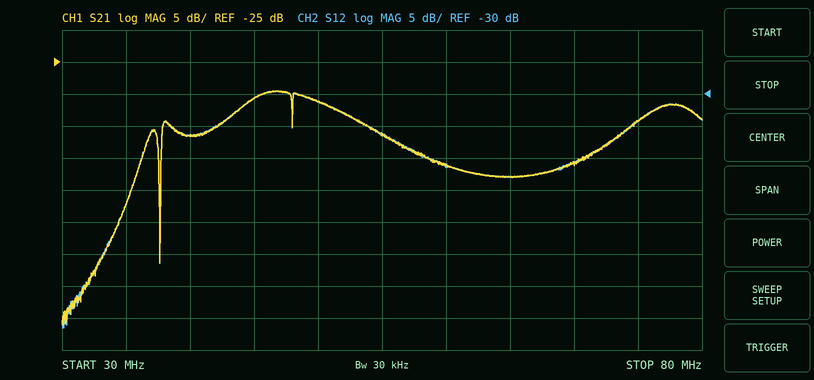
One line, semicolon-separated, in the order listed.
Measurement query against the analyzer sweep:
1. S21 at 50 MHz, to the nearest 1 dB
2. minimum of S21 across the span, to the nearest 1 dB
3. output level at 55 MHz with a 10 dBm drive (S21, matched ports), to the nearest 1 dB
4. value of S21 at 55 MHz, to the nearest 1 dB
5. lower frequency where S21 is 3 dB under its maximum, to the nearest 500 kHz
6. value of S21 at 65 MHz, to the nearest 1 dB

-31 dB; -66 dB; -26 dBm; -36 dB; 44.0 MHz; -43 dB
